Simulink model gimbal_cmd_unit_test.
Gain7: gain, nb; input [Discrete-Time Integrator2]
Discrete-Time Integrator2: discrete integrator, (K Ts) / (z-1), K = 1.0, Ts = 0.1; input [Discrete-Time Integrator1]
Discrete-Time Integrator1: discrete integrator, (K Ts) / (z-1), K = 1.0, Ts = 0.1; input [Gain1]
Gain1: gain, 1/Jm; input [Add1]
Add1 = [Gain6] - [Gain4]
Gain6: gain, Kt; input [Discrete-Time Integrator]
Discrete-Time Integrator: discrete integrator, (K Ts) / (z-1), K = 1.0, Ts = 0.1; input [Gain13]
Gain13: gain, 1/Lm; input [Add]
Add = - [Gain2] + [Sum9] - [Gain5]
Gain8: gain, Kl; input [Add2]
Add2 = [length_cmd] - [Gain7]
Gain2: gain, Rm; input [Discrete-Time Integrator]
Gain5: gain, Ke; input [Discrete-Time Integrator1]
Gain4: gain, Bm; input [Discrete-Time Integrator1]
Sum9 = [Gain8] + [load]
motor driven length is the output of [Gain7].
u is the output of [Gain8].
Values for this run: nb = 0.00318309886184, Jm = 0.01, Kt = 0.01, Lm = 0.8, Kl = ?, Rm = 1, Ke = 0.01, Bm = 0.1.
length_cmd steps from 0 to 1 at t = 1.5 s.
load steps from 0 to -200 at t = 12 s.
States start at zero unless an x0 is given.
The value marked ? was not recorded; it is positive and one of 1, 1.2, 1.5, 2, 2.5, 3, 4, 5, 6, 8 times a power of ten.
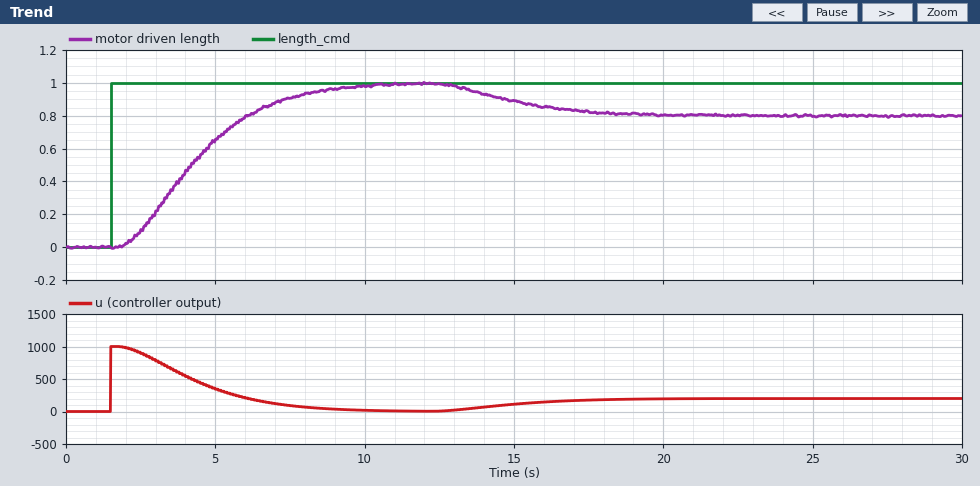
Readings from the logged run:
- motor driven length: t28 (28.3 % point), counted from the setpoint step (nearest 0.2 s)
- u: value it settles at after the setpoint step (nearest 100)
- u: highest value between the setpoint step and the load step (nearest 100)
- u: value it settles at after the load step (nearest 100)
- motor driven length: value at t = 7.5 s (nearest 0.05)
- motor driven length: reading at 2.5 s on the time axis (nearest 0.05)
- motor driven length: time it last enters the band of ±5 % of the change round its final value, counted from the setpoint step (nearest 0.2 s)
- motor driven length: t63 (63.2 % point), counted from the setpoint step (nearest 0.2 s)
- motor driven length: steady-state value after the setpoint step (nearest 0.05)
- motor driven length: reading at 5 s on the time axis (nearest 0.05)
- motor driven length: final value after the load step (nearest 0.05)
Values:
1.8 s
0
1000
200
0.90
0.10
7.0 s
3.4 s
1.00
0.65
0.80
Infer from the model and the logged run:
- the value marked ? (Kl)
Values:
1000
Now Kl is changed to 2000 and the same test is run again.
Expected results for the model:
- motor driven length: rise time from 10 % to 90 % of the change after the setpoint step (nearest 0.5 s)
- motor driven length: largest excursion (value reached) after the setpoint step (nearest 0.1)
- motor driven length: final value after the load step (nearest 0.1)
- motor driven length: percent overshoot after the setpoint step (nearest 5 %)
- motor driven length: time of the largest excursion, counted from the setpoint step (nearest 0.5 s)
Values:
2.0 s
1.1
0.9
10 %
4.5 s
